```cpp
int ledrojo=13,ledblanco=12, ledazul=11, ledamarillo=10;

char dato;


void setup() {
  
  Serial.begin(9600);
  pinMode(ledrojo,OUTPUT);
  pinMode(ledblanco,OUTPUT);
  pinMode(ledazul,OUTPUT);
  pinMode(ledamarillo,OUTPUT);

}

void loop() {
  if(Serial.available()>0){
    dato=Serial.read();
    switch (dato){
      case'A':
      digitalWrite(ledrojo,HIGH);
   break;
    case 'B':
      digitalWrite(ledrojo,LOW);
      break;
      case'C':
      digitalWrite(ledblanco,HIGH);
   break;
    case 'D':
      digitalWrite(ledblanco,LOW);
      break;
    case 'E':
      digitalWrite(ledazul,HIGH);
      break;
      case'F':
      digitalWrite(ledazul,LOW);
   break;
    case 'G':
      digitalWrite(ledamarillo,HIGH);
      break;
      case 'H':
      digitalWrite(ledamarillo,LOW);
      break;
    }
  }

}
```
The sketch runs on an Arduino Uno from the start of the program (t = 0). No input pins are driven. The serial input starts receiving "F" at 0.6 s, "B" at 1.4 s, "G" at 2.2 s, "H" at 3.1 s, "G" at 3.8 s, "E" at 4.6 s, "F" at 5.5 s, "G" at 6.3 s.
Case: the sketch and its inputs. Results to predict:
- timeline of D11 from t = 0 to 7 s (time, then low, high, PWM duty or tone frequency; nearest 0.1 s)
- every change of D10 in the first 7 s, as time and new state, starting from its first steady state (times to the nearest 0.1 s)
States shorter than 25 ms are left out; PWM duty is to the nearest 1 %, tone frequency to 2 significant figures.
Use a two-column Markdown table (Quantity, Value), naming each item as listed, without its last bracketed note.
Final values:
| Quantity | Value |
|---|---|
| timeline of D11 from t = 0 to 7 s | 0 s low; 4.6 s high; 5.5 s low |
| every change of D10 in the first 7 s, as time and new state, starting from its first steady state | 0 s low; 2.2 s high; 3.1 s low; 3.8 s high |
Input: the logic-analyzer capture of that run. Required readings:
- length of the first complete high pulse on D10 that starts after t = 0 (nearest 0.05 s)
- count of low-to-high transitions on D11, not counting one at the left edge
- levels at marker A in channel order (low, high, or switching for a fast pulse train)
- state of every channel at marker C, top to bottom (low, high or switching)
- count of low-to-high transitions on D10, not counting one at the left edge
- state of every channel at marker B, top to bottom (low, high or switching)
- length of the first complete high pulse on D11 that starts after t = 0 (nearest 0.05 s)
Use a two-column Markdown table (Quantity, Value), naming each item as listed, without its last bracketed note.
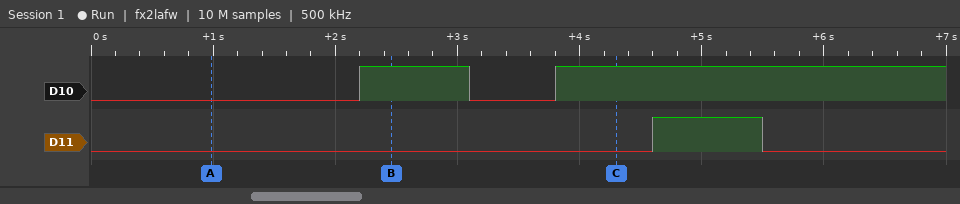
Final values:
| Quantity | Value |
|---|---|
| length of the first complete high pulse on D10 that starts after t = 0 | 0.90 s |
| count of low-to-high transitions on D11, not counting one at the left edge | 1 |
| levels at marker A in channel order | D10 low, D11 low |
| state of every channel at marker C, top to bottom | D10 high, D11 low |
| count of low-to-high transitions on D10, not counting one at the left edge | 2 |
| state of every channel at marker B, top to bottom | D10 high, D11 low |
| length of the first complete high pulse on D11 that starts after t = 0 | 0.90 s |
